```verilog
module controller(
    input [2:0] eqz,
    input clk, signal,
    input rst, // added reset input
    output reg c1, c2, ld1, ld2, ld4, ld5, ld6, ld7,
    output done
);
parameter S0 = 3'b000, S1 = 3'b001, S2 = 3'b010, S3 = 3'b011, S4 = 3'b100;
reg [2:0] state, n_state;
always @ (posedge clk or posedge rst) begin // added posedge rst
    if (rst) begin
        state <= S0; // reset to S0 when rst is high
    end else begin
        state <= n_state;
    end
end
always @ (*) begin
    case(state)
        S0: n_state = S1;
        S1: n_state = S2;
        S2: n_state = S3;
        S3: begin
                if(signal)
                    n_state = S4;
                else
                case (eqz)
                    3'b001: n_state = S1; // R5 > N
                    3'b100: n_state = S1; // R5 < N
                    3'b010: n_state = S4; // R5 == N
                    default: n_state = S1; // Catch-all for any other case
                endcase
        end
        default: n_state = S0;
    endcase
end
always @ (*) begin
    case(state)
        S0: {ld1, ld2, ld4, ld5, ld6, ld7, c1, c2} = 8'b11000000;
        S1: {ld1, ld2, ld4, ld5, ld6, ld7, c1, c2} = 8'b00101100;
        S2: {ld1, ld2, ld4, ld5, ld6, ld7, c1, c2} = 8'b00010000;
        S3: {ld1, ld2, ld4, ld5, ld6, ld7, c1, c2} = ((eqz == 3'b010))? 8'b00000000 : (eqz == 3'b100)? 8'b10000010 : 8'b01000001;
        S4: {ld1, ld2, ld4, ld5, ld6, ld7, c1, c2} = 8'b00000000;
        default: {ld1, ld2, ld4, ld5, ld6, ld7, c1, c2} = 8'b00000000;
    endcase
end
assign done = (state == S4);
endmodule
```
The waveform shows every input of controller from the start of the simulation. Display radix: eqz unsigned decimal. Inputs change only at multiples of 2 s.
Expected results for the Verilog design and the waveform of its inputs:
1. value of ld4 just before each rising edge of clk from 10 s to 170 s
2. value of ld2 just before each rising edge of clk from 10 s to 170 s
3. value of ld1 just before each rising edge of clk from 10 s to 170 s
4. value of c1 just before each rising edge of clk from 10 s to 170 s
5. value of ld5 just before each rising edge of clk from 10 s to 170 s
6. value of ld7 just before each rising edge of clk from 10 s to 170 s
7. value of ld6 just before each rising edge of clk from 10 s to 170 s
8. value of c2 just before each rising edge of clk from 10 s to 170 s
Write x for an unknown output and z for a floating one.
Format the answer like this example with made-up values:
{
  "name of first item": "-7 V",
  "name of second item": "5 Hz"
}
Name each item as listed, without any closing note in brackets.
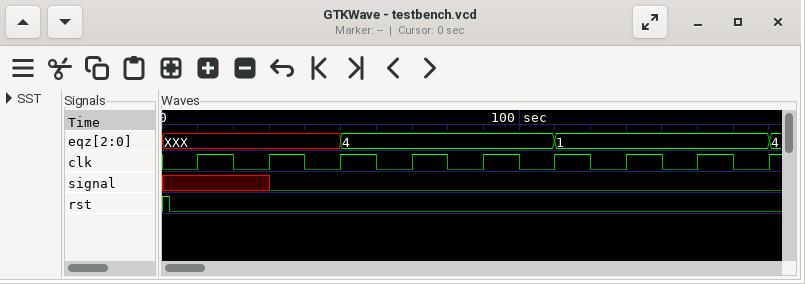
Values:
{
  "value of ld4 just before each rising edge of clk from 10 s to 170 s": "0 1 0 0 1 0 0 1 0",
  "value of ld2 just before each rising edge of clk from 10 s to 170 s": "1 0 0 0 0 0 1 0 0",
  "value of ld1 just before each rising edge of clk from 10 s to 170 s": "1 0 0 1 0 0 0 0 0",
  "value of c1 just before each rising edge of clk from 10 s to 170 s": "0 0 0 1 0 0 0 0 0",
  "value of ld5 just before each rising edge of clk from 10 s to 170 s": "0 0 1 0 0 1 0 0 1",
  "value of ld7 just before each rising edge of clk from 10 s to 170 s": "0 1 0 0 1 0 0 1 0",
  "value of ld6 just before each rising edge of clk from 10 s to 170 s": "0 1 0 0 1 0 0 1 0",
  "value of c2 just before each rising edge of clk from 10 s to 170 s": "0 0 0 0 0 0 1 0 0"
}
